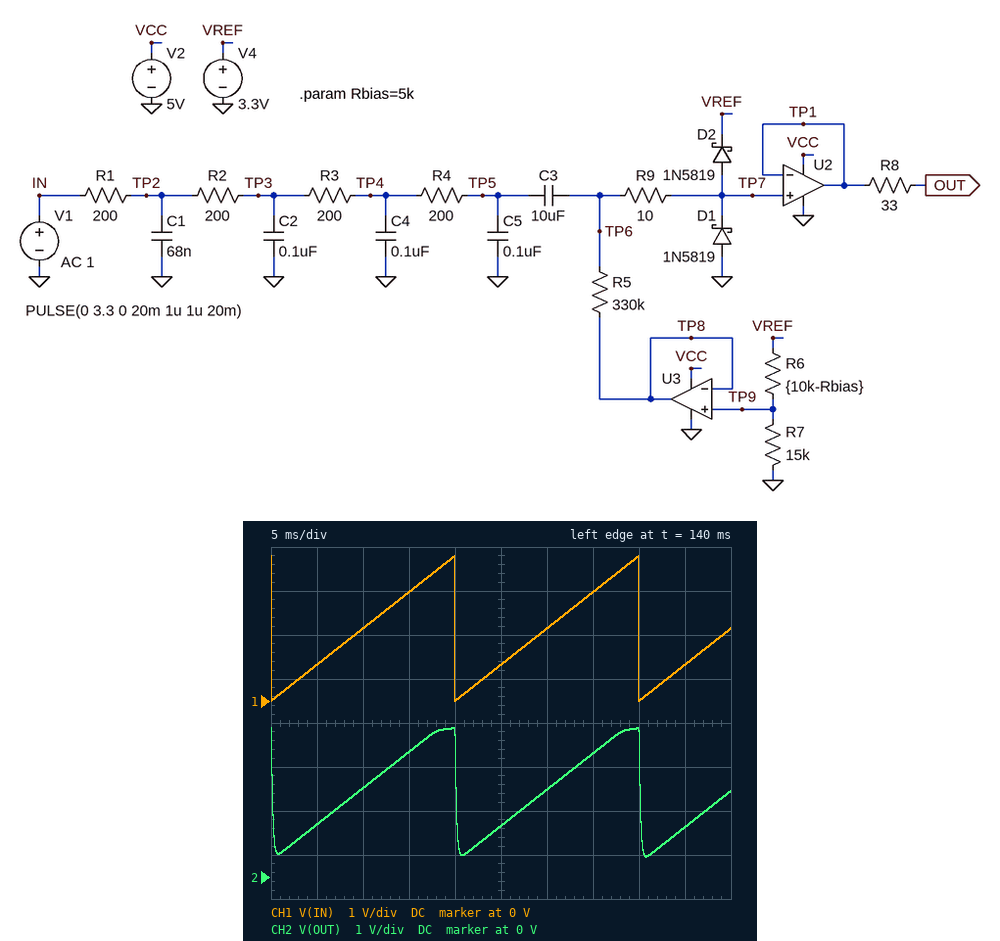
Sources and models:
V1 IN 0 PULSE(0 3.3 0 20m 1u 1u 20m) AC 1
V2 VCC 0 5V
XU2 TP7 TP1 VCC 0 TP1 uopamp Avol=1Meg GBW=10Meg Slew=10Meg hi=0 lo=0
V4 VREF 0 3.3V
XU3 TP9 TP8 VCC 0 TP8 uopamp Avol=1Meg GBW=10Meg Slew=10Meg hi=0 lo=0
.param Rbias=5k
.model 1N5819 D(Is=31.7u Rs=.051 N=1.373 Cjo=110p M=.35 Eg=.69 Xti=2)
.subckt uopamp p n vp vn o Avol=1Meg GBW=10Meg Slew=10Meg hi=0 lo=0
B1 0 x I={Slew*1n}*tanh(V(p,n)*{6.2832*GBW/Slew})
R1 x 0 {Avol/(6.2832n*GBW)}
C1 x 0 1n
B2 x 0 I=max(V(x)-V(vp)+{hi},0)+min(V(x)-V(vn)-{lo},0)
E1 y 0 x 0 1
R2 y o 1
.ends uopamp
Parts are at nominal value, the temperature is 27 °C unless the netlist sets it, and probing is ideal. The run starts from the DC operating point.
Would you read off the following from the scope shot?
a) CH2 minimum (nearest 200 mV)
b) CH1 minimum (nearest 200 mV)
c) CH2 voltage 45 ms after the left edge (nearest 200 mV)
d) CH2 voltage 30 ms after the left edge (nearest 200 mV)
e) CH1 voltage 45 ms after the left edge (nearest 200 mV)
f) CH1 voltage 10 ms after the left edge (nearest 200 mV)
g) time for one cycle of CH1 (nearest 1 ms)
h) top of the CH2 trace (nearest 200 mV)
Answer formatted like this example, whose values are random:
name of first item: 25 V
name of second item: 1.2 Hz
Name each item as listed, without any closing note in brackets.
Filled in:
CH2 minimum: 400 mV
CH1 minimum: 0 V
CH2 voltage 45 ms after the left edge: 1.2 V
CH2 voltage 30 ms after the left edge: 2.0 V
CH1 voltage 45 ms after the left edge: 800 mV
CH1 voltage 10 ms after the left edge: 1.6 V
time for one cycle of CH1: 20 ms
top of the CH2 trace: 3.4 V
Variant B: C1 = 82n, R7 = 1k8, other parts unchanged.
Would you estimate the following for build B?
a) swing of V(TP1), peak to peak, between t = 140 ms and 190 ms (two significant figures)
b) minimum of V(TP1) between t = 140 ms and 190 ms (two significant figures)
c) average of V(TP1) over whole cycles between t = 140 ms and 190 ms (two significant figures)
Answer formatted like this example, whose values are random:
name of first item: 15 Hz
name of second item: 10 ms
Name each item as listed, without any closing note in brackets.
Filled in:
swing of V(TP1), peak to peak, between t = 140 ms and 190 ms: 3.0 V
minimum of V(TP1) between t = 140 ms and 190 ms: 390 mV
average of V(TP1) over whole cycles between t = 140 ms and 190 ms: 1.9 V
